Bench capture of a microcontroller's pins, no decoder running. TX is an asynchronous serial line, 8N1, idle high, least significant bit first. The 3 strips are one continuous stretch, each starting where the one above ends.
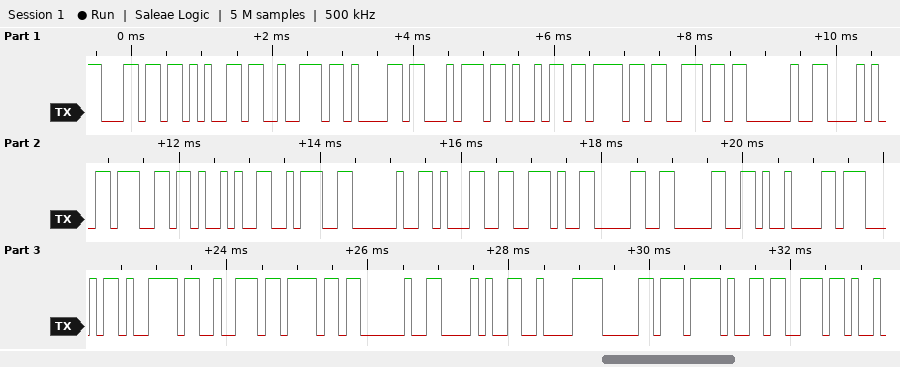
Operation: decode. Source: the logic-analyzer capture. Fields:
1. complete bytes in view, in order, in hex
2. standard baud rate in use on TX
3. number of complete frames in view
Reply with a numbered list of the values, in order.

1. 0x6C 0x65 0x72 0x61 0x74 0x69 0x6F 0x6E 0x20 0x28 0x67 0x29 0x3A 0x20 0x31 0x2E 0x30 0x30 0x09 0x47 0x79 0x72 0x6F 0x20 0x28 0xC2 0xB0 0x2F 0x73
2. 9600 baud
3. 29
